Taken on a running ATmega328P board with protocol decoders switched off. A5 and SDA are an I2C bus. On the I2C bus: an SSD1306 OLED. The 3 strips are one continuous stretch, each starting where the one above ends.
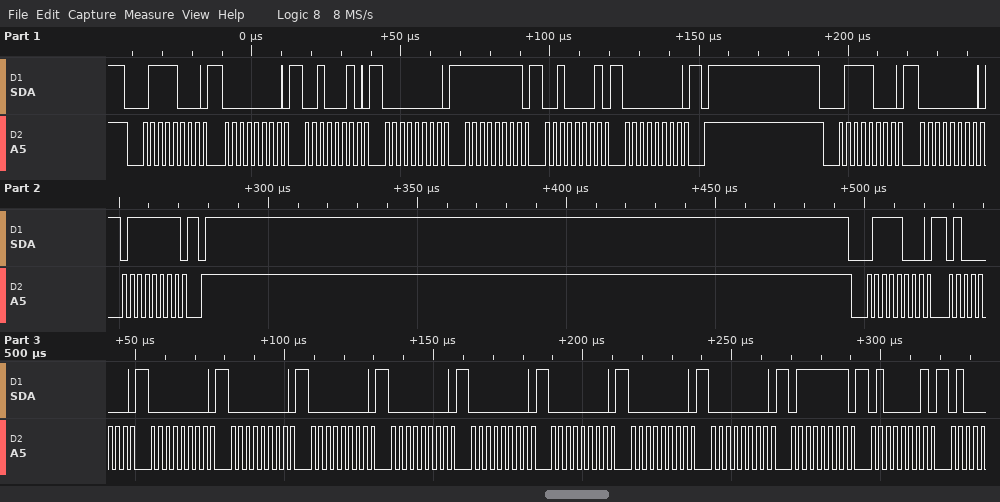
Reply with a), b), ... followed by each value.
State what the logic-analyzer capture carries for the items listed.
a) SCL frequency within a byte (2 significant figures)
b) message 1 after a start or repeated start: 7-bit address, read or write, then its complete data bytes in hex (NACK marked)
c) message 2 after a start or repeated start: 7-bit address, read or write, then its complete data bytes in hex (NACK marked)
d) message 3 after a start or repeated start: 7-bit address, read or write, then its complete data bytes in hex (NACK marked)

a) 400 kHz
b) 0x3C write: 00 22 00 FF 21 00
c) 0x3C write: 00 7F
d) 0x3C write: 40 00 00 00 00 00 00 00 00 7F 41
